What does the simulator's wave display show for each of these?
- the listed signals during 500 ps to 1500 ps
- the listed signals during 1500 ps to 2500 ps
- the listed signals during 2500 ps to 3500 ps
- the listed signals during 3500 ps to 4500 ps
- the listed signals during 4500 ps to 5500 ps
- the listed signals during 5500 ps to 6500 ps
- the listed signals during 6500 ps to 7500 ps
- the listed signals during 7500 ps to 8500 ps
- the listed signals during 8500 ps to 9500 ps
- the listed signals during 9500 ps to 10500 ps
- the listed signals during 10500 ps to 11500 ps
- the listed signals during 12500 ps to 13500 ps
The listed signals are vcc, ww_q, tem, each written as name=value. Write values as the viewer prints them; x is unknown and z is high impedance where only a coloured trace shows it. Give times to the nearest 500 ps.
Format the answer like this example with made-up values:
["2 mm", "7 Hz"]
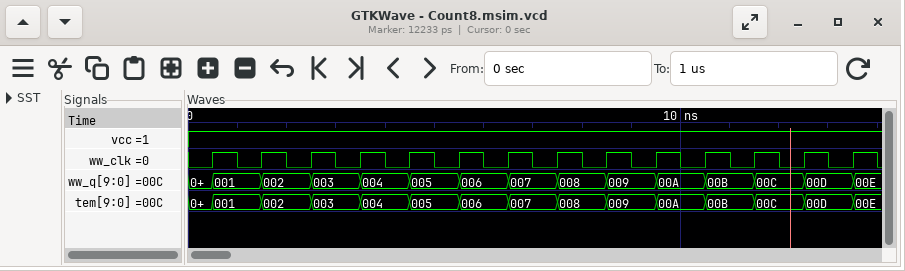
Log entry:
["vcc=1, ww_q=001, tem=001", "vcc=1, ww_q=002, tem=002", "vcc=1, ww_q=003, tem=003", "vcc=1, ww_q=004, tem=004", "vcc=1, ww_q=005, tem=005", "vcc=1, ww_q=006, tem=006", "vcc=1, ww_q=007, tem=007", "vcc=1, ww_q=008, tem=008", "vcc=1, ww_q=009, tem=009", "vcc=1, ww_q=00A, tem=00A", "vcc=1, ww_q=00B, tem=00B", "vcc=1, ww_q=00D, tem=00D"]
